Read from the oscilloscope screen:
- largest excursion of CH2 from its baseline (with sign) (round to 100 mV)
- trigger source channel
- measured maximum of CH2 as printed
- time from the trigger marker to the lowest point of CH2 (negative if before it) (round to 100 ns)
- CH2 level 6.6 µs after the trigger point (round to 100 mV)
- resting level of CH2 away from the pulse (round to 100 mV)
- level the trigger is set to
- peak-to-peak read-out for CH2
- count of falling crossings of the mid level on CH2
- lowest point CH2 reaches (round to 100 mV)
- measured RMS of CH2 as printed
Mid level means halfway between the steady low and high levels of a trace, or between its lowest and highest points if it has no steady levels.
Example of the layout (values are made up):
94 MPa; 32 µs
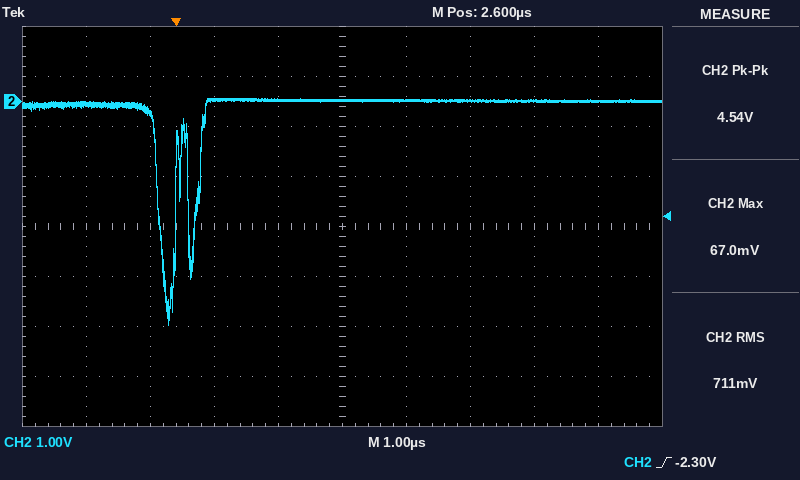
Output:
-4.5 V; CH2; 67.0 mV; -100 ns; 0.0 V; 0.0 V; -2.30 V; 4.54 V; 2; -4.5 V; 711 mV
